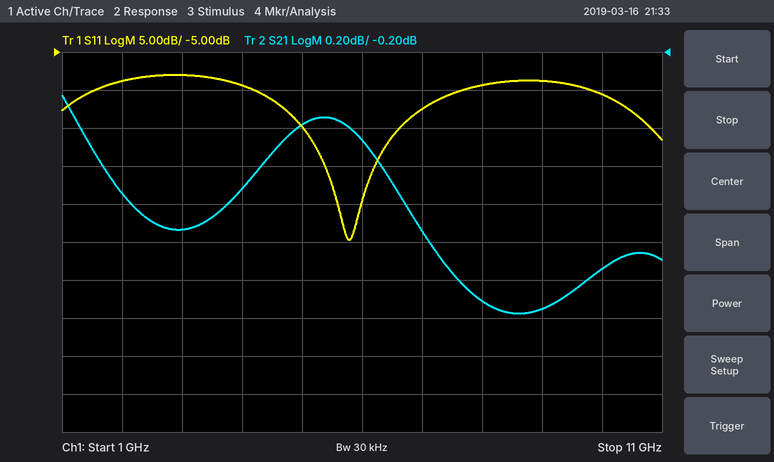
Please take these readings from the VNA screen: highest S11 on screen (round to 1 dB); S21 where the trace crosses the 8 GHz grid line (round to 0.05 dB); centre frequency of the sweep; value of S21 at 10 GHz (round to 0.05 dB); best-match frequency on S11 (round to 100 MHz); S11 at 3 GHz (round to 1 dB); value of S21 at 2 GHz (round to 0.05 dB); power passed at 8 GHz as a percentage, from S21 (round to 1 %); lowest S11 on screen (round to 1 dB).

-8 dB
-1.50 dB
6 GHz
-1.35 dB
5.8 GHz
-8 dB
-0.95 dB
71 %
-30 dB
